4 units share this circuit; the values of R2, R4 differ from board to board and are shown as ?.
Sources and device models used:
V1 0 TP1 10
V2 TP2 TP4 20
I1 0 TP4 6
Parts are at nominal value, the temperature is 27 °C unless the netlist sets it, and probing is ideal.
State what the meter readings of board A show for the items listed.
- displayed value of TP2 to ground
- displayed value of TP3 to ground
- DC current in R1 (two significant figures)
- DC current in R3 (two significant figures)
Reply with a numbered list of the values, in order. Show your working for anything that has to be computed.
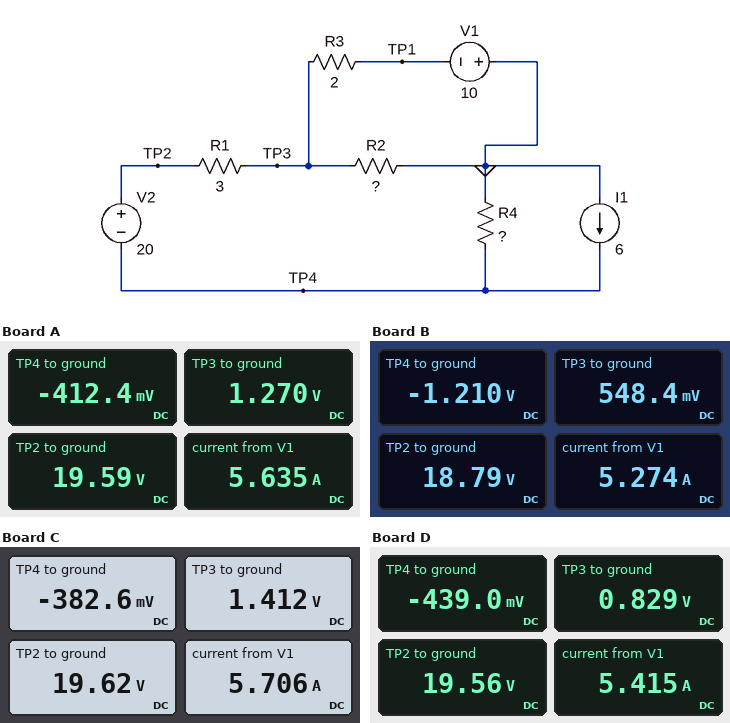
1. 19.59 V
2. 1.270 V
3. (19.59 V - 1.27 V) / 3 Ω = 6.1 A
4. (1.27 V - (-10 V)) / 2 Ω = 5.6 A
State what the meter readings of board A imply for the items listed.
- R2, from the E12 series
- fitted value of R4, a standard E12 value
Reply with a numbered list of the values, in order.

1. 2.7 Ω
2. 3.9 Ω
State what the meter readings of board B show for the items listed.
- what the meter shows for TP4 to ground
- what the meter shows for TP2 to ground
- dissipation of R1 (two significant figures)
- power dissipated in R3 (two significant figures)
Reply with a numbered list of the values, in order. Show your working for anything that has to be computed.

1. -1.210 V
2. 18.79 V
3. (18.79 V - 548.4 mV)^2 / 3 Ω = 110 W
4. (548.4 mV - (-10 V))^2 / 2 Ω = 56 W
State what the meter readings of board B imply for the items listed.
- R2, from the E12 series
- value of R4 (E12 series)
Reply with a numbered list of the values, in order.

1. 0.68 Ω
2. 15 Ω
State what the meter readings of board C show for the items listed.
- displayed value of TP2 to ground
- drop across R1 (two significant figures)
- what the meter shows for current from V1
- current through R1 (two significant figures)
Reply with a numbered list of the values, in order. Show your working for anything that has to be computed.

1. 19.62 V
2. 19.62 V - 1.412 V = 18 V
3. 5.706 A
4. (19.62 V - 1.412 V) / 3 Ω = 6.1 A
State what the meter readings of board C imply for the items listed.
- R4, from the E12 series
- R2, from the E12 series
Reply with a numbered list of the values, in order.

1. 5.6 Ω
2. 3.9 Ω
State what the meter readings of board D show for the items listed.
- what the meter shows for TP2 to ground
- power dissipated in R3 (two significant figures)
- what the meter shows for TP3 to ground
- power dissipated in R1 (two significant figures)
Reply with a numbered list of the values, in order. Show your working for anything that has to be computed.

1. 19.56 V
2. (829 mV - (-10 V))^2 / 2 Ω = 59 W
3. 0.829 V
4. (19.56 V - 829 mV)^2 / 3 Ω = 120 W
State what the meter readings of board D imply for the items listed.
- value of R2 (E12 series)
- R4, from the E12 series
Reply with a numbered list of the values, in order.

1. 1 Ω
2. 1.8 Ω
